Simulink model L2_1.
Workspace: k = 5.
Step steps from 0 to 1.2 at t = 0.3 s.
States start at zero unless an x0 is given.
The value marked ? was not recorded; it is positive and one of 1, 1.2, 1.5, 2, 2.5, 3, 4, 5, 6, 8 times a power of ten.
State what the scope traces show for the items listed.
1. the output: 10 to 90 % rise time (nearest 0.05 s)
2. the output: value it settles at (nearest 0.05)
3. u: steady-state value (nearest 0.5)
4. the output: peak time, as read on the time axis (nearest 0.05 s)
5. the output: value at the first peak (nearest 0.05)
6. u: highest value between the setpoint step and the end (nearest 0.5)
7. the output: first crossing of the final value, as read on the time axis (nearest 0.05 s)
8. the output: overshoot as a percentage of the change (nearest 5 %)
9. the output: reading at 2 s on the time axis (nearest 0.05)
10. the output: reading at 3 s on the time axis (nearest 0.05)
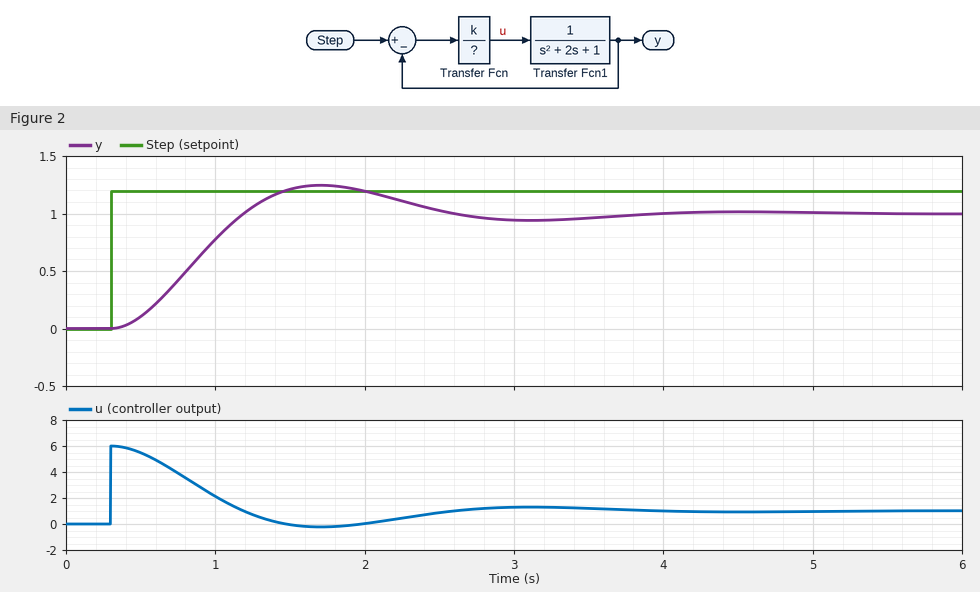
0.60 s
1.00
1.0
1.70 s
1.25
6.0
1.20 s
25 %
1.20
0.95
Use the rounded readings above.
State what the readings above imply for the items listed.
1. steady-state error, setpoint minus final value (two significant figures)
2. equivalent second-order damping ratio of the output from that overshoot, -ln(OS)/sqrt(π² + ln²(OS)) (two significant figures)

0.20
0.40
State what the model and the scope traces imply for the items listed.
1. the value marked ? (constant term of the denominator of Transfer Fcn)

1
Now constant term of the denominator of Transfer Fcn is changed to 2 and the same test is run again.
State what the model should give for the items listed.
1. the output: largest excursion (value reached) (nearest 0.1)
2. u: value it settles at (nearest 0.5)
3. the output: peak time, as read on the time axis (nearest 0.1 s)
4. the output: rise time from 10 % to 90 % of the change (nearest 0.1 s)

1.0
1.0
2.3 s
0.9 s
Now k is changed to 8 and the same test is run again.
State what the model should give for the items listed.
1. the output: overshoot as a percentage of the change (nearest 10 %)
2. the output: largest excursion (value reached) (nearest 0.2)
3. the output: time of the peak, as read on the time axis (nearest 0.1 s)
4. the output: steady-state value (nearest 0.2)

30 %
1.4
1.4 s
1.0
